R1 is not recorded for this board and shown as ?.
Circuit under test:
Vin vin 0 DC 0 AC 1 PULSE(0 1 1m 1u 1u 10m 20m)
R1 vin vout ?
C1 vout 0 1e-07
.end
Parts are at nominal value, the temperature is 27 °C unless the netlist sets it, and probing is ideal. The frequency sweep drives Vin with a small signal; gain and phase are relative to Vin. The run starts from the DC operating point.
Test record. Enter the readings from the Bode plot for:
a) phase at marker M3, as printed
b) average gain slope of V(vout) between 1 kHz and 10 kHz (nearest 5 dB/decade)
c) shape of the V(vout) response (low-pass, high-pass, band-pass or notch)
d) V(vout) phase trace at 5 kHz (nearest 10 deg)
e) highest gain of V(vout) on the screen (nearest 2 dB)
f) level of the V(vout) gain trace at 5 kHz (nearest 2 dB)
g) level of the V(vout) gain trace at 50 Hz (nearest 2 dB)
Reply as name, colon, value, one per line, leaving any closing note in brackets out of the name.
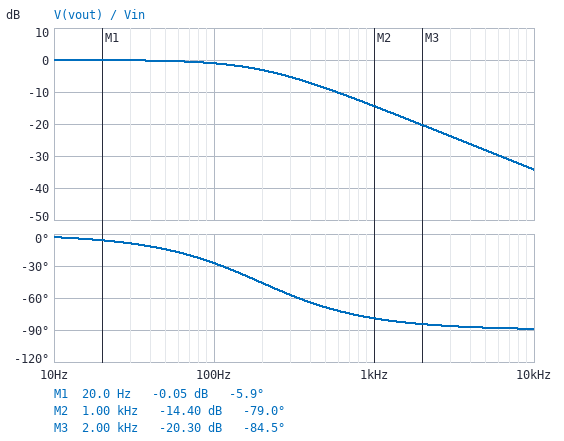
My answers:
phase at marker M3, as printed: -84.5 deg
average gain slope of V(vout) between 1 kHz and 10 kHz: -20 dB/decade
shape of the V(vout) response: low-pass
V(vout) phase trace at 5 kHz: -90 deg
highest gain of V(vout) on the screen: 0 dB
level of the V(vout) gain trace at 5 kHz: -28 dB
level of the V(vout) gain trace at 50 Hz: 0 dB
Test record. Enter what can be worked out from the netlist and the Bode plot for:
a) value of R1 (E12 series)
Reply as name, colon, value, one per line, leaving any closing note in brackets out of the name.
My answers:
value of R1: 8.2 kΩ
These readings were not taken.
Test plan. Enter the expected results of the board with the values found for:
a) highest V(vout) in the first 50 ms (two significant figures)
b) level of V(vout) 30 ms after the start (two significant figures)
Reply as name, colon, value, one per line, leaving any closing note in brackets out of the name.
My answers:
highest V(vout) in the first 50 ms: 1.0 V
level of V(vout) 30 ms after the start: 1.0 V
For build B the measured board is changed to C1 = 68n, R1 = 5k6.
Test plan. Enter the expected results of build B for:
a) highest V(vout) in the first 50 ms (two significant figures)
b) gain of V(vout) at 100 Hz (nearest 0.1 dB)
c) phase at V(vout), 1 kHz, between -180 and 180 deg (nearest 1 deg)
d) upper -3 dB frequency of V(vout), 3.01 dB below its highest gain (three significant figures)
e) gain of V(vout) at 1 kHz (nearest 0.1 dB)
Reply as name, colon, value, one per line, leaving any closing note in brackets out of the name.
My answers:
highest V(vout) in the first 50 ms: 1.0 V
gain of V(vout) at 100 Hz: -0.2 dB
phase at V(vout), 1 kHz, between -180 and 180 deg: -67 deg
upper -3 dB frequency of V(vout), 3.01 dB below its highest gain: 418 Hz
gain of V(vout) at 1 kHz: -8.3 dB
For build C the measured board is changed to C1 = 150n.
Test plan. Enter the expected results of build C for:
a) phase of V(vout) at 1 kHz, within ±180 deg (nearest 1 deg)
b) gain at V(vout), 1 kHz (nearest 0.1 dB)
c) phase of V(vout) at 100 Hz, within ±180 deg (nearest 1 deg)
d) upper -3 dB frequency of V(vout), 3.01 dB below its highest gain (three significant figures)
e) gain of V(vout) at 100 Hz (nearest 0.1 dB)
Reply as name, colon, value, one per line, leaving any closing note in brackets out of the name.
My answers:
phase of V(vout) at 1 kHz, within ±180 deg: -83 deg
gain at V(vout), 1 kHz: -17.8 dB
phase of V(vout) at 100 Hz, within ±180 deg: -38 deg
upper -3 dB frequency of V(vout), 3.01 dB below its highest gain: 129 Hz
gain of V(vout) at 100 Hz: -2.0 dB
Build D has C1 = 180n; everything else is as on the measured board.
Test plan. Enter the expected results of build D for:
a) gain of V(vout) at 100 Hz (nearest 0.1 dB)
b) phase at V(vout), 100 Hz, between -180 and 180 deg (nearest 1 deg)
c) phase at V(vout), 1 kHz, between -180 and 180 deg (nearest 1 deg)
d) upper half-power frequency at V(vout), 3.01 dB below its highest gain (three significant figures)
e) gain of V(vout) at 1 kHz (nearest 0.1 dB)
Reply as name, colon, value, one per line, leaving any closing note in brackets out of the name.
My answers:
gain of V(vout) at 100 Hz: -2.7 dB
phase at V(vout), 100 Hz, between -180 and 180 deg: -43 deg
phase at V(vout), 1 kHz, between -180 and 180 deg: -84 deg
upper half-power frequency at V(vout), 3.01 dB below its highest gain: 108 Hz
gain of V(vout) at 1 kHz: -19.4 dB
